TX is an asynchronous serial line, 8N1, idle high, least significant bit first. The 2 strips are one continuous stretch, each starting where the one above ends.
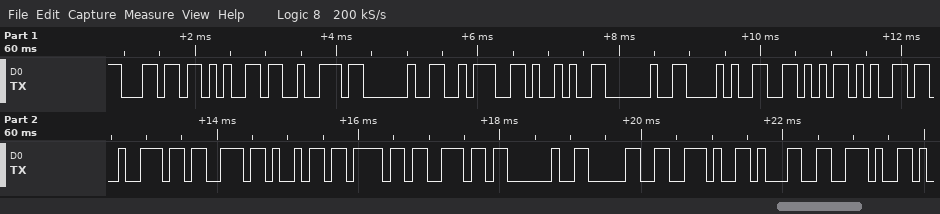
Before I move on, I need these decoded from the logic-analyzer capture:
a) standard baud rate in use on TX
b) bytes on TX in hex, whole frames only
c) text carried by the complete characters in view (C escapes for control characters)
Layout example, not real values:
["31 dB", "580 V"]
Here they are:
["9600 baud", "6C 65 72 20 3A 29 20 28 56 65 72 73 69 6F 6E 20 30 2E 31 2E", "\"ler :) (Version 0.1.\""]
